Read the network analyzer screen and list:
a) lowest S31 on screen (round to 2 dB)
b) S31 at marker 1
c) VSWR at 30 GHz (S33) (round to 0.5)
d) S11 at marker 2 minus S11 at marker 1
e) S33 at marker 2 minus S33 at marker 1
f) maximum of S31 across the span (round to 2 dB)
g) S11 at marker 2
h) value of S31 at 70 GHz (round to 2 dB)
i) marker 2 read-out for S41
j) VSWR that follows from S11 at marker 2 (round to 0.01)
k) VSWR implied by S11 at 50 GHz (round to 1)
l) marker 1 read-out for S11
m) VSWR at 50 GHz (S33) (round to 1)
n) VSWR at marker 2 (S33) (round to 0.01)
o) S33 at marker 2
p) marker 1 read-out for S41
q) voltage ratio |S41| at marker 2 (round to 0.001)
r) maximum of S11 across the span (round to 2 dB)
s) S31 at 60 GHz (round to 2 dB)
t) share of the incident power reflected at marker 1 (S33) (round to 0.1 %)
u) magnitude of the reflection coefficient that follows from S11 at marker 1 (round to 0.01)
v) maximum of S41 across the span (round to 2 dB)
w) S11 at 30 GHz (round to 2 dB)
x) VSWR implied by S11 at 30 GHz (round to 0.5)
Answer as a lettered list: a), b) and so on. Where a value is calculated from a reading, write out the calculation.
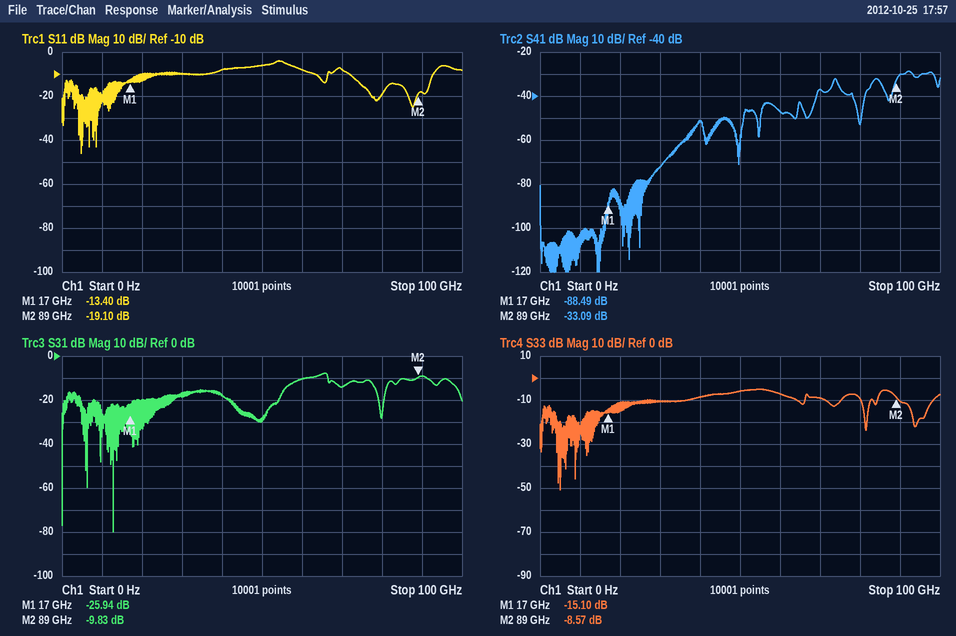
a) -80 dB
b) -25.94 dB
c) |Γ| = 10^(-10/20) = 0.3162; VSWR = (1 + 0.3162)/(1 − 0.3162) ≈ 1.92, so 2.0 to the nearest 0.5
d) -19.1 − (-13.4) = -5.70 dB
e) -8.57 − (-15.1) = 6.53 dB
f) -8 dB
g) -19.10 dB
h) -14 dB
i) -33.09 dB
j) (1 + 0.1109)/(1 − 0.1109) ≈ 1.25
k) |Γ| = 10^(-6/20) = 0.5012; VSWR = (1 + 0.5012)/(1 − 0.5012) ≈ 3
l) -13.40 dB
m) |Γ| = 10^(-6/20) = 0.5012; VSWR = (1 + 0.5012)/(1 − 0.5012) ≈ 3
n) (1 + 0.3728)/(1 − 0.3728) ≈ 2.19
o) -8.57 dB
p) -88.49 dB
q) 10^(-33.09/20) ≈ 0.022
r) -4 dB
s) -10 dB
t) 10^(-15.1/10) ≈ 3.1 %
u) 10^(-13.4/20) ≈ 0.21
v) -28 dB
w) -10 dB
x) |Γ| = 10^(-10/20) = 0.3162; VSWR = (1 + 0.3162)/(1 − 0.3162) ≈ 1.92, so 2.0 to the nearest 0.5
